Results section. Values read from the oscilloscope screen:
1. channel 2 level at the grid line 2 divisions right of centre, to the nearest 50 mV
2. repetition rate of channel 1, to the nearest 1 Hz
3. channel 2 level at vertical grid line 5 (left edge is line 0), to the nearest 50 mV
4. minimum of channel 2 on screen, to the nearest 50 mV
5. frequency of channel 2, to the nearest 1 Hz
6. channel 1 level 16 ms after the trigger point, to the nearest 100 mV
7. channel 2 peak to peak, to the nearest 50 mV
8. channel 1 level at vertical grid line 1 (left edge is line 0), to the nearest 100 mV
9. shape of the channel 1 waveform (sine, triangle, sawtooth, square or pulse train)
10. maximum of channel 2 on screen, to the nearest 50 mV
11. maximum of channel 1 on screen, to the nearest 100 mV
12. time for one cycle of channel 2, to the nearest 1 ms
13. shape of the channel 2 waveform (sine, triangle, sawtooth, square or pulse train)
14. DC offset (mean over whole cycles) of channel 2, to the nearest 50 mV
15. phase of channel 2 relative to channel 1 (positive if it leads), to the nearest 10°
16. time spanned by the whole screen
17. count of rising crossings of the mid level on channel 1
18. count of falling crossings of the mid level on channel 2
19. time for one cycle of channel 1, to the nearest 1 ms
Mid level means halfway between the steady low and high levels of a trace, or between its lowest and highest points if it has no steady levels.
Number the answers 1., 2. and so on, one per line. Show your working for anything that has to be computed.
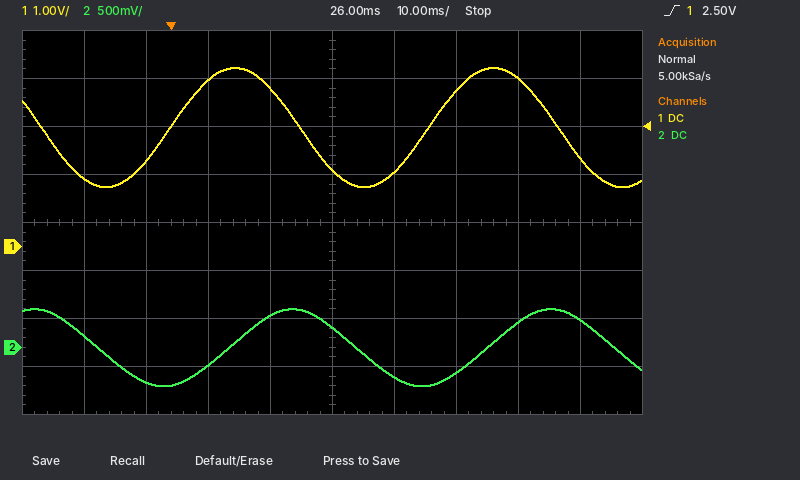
1. -250 mV
2. 1 / 42 ms ≈ 24 Hz
3. 200 mV
4. -400 mV
5. 1 / 42 ms ≈ 24 Hz
6. 3.3 V
7. 400 mV − (-400 mV) = 800 mV
8. 1.4 V
9. sine
10. 400 mV
11. 3.7 V
12. 42 ms
13. sine
14. (400 mV + (-400 mV)) / 2 ≈ 0 mV
15. -80°
16. 100 ms
17. 2
18. 3
19. 42 ms
